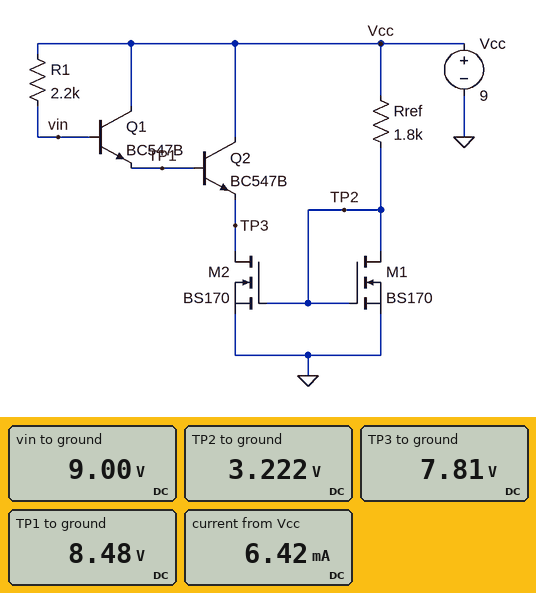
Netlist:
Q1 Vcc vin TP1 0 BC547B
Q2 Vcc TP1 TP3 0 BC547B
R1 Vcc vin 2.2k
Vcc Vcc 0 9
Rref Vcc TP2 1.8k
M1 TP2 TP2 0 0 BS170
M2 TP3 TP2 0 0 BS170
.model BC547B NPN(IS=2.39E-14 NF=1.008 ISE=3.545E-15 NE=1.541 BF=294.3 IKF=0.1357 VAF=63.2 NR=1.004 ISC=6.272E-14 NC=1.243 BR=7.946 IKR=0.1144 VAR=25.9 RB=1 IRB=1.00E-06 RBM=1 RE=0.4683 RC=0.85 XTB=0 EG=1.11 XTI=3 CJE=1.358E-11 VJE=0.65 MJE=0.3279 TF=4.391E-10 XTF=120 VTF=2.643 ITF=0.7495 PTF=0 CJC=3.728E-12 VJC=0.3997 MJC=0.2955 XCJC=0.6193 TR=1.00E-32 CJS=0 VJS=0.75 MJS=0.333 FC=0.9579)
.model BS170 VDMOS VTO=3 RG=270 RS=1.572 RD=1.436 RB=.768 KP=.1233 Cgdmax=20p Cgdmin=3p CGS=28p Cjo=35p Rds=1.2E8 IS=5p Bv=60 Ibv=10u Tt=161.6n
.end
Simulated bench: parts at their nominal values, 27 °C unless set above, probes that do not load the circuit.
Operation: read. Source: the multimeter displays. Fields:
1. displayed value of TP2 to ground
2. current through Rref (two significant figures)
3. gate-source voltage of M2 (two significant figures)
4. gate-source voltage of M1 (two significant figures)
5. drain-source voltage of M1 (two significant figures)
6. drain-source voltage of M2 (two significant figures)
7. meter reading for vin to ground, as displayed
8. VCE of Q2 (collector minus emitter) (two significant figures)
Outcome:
3.222 V
3.2 mA
3.2 V
3.2 V
3.2 V
7.8 V
9.00 V
1.2 V
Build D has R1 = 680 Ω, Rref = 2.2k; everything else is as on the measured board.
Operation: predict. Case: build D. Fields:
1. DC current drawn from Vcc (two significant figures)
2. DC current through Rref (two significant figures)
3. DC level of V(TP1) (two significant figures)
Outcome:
5.3 mA
2.6 mA
8.5 V
